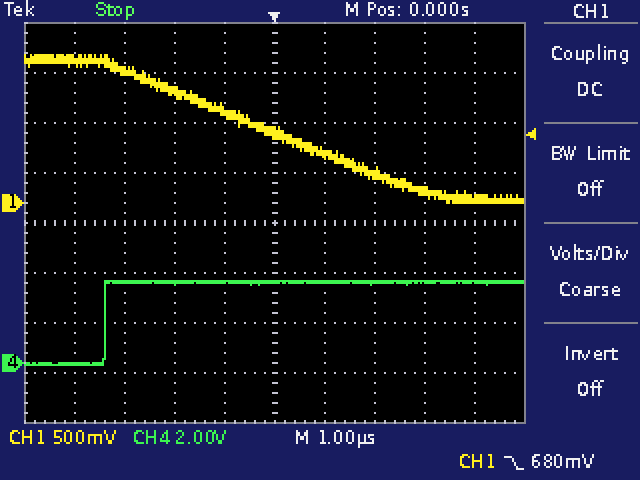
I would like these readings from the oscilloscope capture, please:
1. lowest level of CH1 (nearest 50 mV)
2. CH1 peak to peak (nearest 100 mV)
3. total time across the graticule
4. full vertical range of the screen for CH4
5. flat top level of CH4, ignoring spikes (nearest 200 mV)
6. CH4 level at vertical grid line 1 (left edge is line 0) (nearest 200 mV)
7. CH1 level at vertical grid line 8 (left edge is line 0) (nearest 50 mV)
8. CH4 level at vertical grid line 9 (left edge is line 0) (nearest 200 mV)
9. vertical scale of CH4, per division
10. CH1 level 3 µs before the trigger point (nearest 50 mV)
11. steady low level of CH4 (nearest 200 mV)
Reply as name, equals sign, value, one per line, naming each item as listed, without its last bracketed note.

lowest level of CH1 = 0 mV
CH1 peak to peak = 1.50 V
total time across the graticule = 10 µs
full vertical range of the screen for CH4 = 16 V
flat top level of CH4, ignoring spikes = 3.2 V
CH4 level at vertical grid line 1 (left edge is line 0) = 0.0 V
CH1 level at vertical grid line 8 (left edge is line 0) = 100 mV
CH4 level at vertical grid line 9 (left edge is line 0) = 3.2 V
vertical scale of CH4, per division = 2 V
CH1 level 3 µs before the trigger point = 1.30 V
steady low level of CH4 = 0.0 V
